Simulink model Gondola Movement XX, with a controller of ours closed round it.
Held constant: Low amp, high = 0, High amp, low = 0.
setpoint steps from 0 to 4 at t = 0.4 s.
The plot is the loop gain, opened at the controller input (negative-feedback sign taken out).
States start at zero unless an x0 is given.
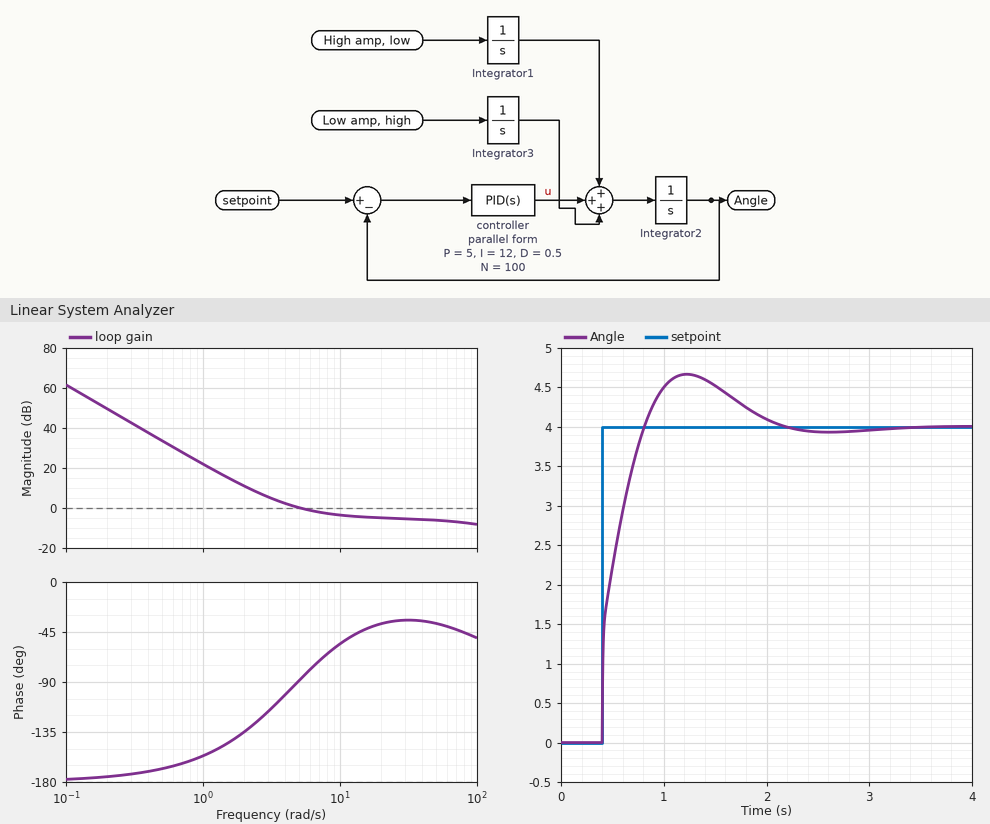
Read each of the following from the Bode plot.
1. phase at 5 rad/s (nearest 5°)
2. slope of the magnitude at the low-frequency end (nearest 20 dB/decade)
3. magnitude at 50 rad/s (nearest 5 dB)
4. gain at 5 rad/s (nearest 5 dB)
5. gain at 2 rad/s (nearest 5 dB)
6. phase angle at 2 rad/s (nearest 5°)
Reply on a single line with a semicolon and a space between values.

-90°; -40 dB/decade; -5 dB; 0 dB; 10 dB; -135°
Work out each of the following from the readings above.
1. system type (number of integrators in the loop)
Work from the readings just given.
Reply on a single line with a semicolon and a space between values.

2
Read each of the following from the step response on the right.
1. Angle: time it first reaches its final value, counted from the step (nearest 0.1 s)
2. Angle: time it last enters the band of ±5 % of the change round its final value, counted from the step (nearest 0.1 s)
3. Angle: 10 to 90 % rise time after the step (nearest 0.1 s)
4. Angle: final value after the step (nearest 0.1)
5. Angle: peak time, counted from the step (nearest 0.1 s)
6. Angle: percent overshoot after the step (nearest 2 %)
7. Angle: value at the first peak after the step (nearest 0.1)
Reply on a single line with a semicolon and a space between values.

0.4 s; 1.5 s; 0.3 s; 4.0; 0.8 s; 16 %; 4.7
